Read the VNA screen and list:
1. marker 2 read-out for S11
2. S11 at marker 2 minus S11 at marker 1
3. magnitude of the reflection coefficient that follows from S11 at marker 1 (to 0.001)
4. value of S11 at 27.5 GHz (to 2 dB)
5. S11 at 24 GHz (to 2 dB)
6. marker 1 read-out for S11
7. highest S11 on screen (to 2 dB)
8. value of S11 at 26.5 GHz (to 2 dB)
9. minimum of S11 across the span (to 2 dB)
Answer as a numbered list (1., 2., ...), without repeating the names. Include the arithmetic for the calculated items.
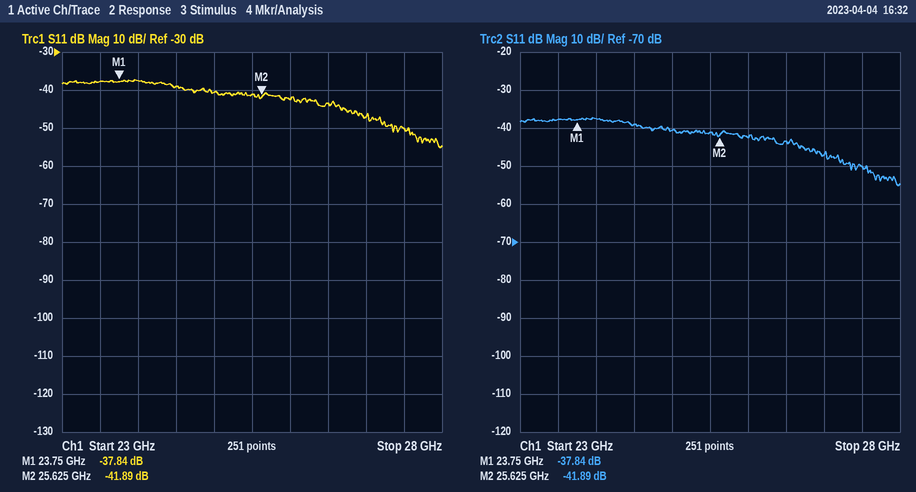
1. -41.89 dB
2. -41.89 − (-37.84) = -4.05 dB
3. 10^(-37.84/20) ≈ 0.013
4. -50 dB
5. -38 dB
6. -37.84 dB
7. -38 dB
8. -44 dB
9. -56 dB
